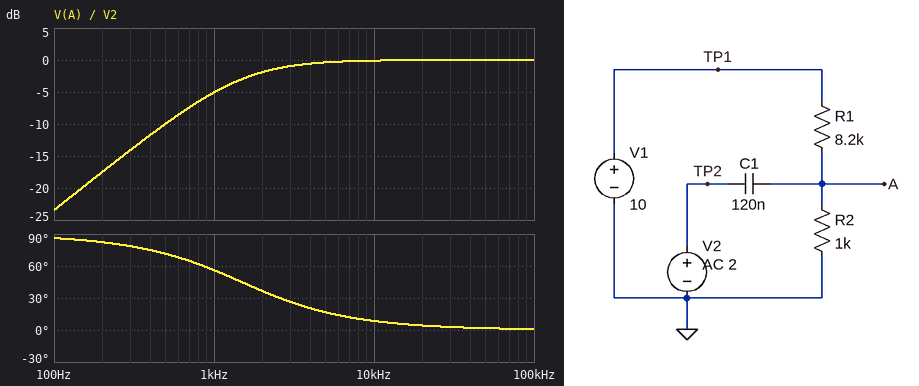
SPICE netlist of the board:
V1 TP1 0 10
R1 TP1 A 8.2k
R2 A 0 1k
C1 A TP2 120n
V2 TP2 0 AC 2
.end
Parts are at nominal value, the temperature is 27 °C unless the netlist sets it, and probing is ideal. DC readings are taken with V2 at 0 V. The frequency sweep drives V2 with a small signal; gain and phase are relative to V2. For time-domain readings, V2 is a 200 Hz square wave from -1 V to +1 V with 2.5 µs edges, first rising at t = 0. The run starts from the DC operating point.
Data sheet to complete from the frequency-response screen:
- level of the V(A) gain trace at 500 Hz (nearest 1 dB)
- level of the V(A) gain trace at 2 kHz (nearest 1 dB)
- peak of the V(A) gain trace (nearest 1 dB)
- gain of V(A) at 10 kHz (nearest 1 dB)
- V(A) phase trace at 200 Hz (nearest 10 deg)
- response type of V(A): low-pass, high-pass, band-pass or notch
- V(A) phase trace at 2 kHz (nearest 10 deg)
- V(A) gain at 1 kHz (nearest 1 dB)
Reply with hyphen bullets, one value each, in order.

- -10 dB
- -2 dB
- 0 dB
- 0 dB
- 80 deg
- high-pass
- 40 deg
- -5 dB
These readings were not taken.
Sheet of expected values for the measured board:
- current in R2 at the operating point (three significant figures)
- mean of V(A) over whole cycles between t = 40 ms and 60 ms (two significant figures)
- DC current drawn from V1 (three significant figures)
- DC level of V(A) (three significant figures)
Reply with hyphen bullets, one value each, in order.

- 1.09 mA
- 1.1 V
- 1.09 mA
- 1.09 V
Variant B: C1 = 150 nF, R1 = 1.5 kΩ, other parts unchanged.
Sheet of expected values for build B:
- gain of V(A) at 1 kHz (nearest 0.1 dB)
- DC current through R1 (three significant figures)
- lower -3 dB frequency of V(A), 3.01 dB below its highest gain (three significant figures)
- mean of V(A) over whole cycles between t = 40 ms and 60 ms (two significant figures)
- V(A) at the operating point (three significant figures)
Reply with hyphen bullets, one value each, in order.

- -6.2 dB
- 4.00 mA
- 1.77 kHz
- 4.0 V
- 4.00 V
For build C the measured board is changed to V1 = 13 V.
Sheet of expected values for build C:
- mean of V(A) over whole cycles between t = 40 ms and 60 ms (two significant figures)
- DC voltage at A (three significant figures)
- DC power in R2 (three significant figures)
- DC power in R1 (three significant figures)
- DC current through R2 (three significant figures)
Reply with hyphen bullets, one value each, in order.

- 1.4 V
- 1.41 V
- 2.00 mW
- 16.4 mW
- 1.41 mA
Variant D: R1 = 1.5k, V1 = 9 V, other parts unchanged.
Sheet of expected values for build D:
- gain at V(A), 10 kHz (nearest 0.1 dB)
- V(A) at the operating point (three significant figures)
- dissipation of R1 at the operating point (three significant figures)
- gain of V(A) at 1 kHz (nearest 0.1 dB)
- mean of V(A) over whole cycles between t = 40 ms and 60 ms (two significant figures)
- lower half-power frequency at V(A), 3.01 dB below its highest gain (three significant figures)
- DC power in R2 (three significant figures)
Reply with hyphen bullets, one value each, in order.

- -0.2 dB
- 3.60 V
- 19.4 mW
- -7.7 dB
- 3.6 V
- 2.21 kHz
- 13.0 mW
